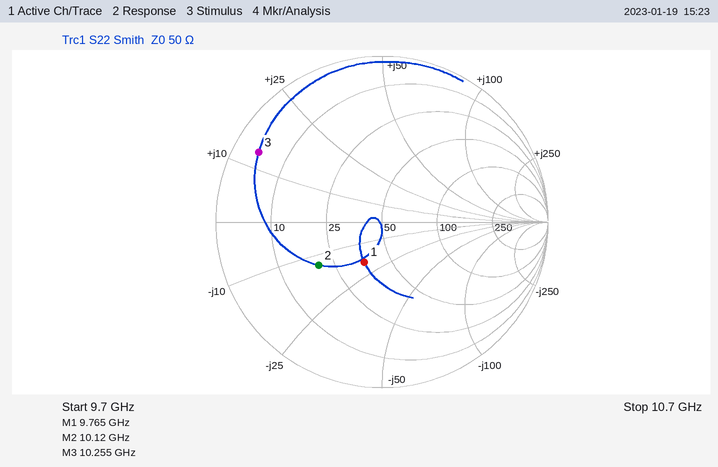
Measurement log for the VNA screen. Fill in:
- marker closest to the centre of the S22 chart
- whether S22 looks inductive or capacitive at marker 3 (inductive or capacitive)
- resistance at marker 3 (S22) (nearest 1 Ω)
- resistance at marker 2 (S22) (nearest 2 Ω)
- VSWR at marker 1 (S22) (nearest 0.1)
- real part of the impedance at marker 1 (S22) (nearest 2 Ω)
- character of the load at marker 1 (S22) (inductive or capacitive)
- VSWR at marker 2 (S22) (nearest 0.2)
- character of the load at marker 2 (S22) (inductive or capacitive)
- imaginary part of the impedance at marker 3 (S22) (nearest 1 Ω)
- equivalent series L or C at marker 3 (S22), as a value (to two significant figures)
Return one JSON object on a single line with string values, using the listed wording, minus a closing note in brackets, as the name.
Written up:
{"marker closest to the centre of the S22 chart": "marker 1", "whether S22 looks inductive or capacitive at marker 3": "inductive", "resistance at marker 3 (S22)": "4 Ω", "resistance at marker 2 (S22)": "20 Ω", "VSWR at marker 1 (S22)": "1.7", "real part of the impedance at marker 1 (S22)": "36 Ω", "character of the load at marker 1 (S22)": "capacitive", "VSWR at marker 2 (S22)": "2.8", "character of the load at marker 2 (S22)": "capacitive", "imaginary part of the impedance at marker 3 (S22)": "+13 Ω", "equivalent series L or C at marker 3 (S22), as a value": "200 pH"}
